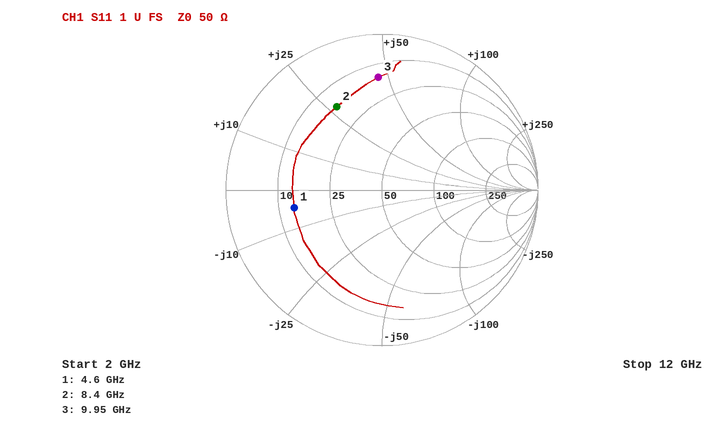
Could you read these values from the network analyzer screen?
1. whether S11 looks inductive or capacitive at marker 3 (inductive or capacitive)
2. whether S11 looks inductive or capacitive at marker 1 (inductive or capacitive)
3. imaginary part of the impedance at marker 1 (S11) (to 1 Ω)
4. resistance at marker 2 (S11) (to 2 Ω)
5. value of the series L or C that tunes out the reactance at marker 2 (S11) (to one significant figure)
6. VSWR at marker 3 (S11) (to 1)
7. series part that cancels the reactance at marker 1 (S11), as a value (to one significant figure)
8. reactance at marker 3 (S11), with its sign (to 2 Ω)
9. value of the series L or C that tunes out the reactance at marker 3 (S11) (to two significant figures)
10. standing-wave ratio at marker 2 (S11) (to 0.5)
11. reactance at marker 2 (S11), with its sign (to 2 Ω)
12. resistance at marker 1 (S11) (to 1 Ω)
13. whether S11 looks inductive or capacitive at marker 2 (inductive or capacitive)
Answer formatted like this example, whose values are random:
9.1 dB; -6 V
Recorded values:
inductive; capacitive; -5 Ω; 16 Ω; 700 fF; 6; 200 pH; +46 Ω; 350 fF; 4.0; +28 Ω; 14 Ω; inductive
